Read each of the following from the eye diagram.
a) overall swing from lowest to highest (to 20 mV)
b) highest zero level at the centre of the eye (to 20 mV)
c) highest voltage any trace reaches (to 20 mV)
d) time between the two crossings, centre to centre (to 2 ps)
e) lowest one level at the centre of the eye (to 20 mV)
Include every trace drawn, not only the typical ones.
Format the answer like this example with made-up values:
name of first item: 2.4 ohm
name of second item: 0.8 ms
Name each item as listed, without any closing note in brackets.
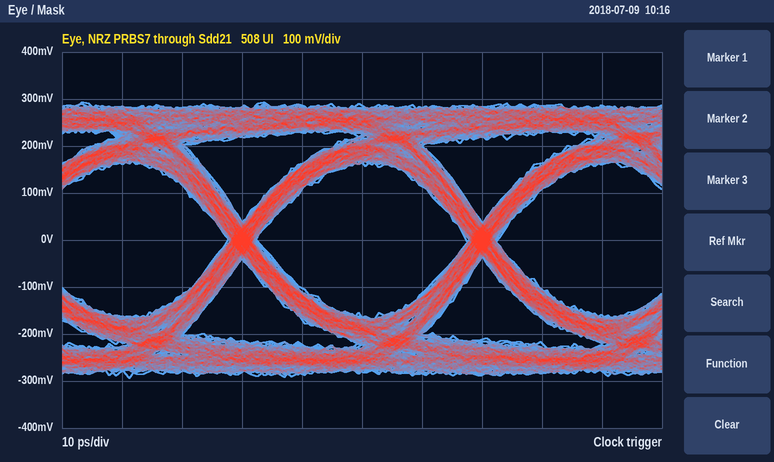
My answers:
overall swing from lowest to highest: 580 mV
highest zero level at the centre of the eye: -160 mV
highest voltage any trace reaches: 300 mV
time between the two crossings, centre to centre: 40 ps
lowest one level at the centre of the eye: 160 mV
